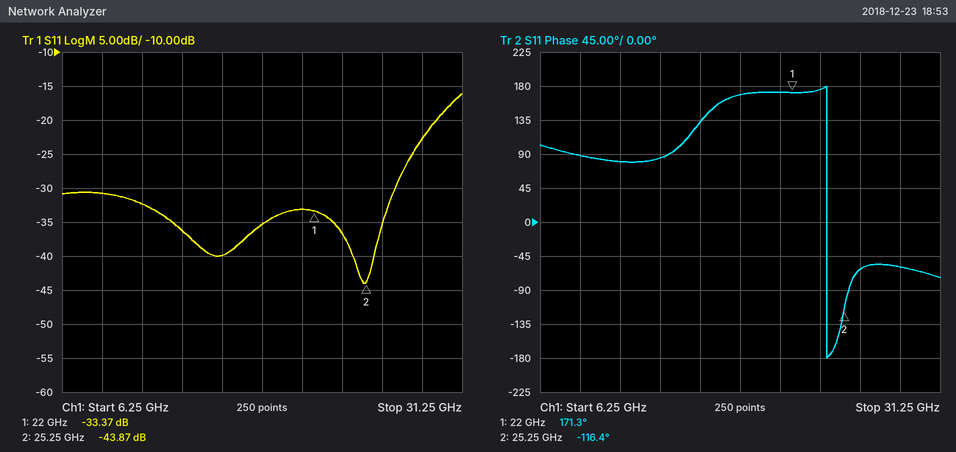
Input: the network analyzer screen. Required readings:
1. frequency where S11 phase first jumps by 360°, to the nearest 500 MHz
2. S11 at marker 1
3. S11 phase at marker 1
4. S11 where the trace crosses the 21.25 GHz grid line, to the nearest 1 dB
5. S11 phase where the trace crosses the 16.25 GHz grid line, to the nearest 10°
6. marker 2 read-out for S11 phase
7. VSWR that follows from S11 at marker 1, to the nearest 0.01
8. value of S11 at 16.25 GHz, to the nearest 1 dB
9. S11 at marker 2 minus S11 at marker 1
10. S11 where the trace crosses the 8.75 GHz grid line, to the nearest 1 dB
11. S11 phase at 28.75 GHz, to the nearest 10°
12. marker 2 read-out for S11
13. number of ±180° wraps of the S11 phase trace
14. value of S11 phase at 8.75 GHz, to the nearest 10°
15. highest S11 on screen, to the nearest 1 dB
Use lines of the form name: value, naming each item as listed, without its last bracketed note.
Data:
frequency where S11 phase first jumps by 360°, to the nearest 500 MHz: 24.0 GHz
S11 at marker 1: -33.37 dB
S11 phase at marker 1: 171.3°
S11 where the trace crosses the 21.25 GHz grid line, to the nearest 1 dB: -33 dB
S11 phase where the trace crosses the 16.25 GHz grid line, to the nearest 10°: 130°
marker 2 read-out for S11 phase: -116.4°
VSWR that follows from S11 at marker 1, to the nearest 0.01: 1.04
value of S11 at 16.25 GHz, to the nearest 1 dB: -40 dB
S11 at marker 2 minus S11 at marker 1: -10.50 dB
S11 where the trace crosses the 8.75 GHz grid line, to the nearest 1 dB: -31 dB
S11 phase at 28.75 GHz, to the nearest 10°: -60°
marker 2 read-out for S11: -43.87 dB
number of ±180° wraps of the S11 phase trace: 1
value of S11 phase at 8.75 GHz, to the nearest 10°: 90°
highest S11 on screen, to the nearest 1 dB: -16 dB
